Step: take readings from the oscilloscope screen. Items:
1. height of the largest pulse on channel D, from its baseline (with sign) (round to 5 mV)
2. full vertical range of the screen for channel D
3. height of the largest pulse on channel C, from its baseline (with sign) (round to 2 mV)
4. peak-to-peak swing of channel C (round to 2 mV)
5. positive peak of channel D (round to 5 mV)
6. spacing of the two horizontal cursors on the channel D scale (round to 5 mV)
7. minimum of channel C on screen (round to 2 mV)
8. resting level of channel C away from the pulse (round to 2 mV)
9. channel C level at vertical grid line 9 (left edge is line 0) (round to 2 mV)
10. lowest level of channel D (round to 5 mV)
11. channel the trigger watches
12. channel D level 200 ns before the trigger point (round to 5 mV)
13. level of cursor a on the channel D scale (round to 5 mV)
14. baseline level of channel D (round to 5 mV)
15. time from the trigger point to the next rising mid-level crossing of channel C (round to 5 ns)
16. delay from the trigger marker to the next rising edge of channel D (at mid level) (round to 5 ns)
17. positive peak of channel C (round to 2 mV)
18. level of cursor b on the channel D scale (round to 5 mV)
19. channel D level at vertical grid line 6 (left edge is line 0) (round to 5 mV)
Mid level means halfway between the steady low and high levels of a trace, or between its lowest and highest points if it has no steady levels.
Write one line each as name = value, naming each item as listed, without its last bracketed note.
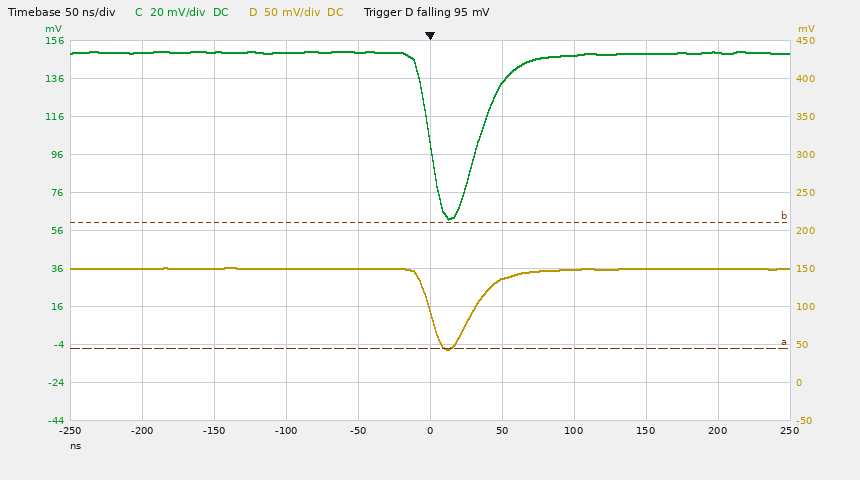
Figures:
height of the largest pulse on channel D, from its baseline (with sign) = -105 mV
full vertical range of the screen for channel D = 500 mV
height of the largest pulse on channel C, from its baseline (with sign) = -88 mV
peak-to-peak swing of channel C = 88 mV
positive peak of channel D = 150 mV
spacing of the two horizontal cursors on the channel D scale = 165 mV
minimum of channel C on screen = 62 mV
resting level of channel C away from the pulse = 150 mV
channel C level at vertical grid line 9 (left edge is line 0) = 150 mV
lowest level of channel D = 45 mV
channel the trigger watches = channel D
channel D level 200 ns before the trigger point = 150 mV
level of cursor a on the channel D scale = 45 mV
baseline level of channel D = 150 mV
time from the trigger point to the next rising mid-level crossing of channel C = 35 ns
delay from the trigger marker to the next rising edge of channel D (at mid level) = 30 ns
positive peak of channel C = 150 mV
level of cursor b on the channel D scale = 210 mV
channel D level at vertical grid line 6 (left edge is line 0) = 135 mV
